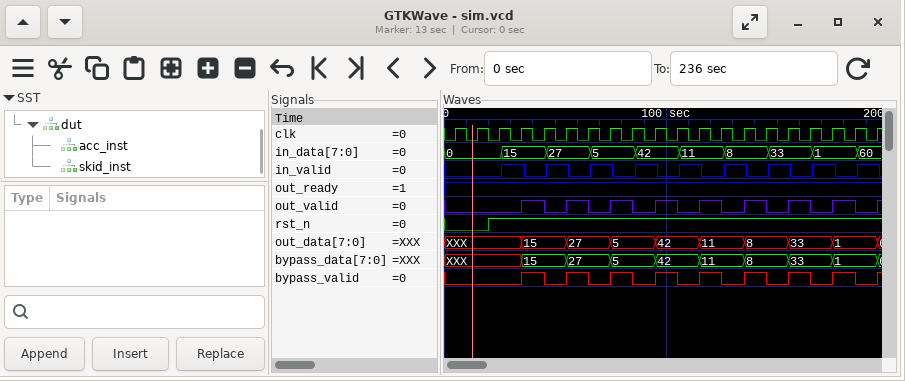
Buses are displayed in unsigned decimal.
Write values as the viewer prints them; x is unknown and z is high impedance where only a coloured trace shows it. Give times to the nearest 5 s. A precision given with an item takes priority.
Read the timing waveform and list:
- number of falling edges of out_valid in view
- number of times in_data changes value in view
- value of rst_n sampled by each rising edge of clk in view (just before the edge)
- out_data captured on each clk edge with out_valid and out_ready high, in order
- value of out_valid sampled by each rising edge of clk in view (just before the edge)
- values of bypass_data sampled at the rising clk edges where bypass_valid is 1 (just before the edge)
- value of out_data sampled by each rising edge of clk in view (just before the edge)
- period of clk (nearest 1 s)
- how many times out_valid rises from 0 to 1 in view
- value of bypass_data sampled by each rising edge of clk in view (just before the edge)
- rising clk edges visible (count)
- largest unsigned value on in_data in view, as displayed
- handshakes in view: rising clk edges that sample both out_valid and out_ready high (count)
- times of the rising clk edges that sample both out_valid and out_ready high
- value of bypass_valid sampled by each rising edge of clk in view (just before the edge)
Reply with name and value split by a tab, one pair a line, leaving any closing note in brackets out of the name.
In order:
number of falling edges of out_valid in view	8
number of times in_data changes value in view	9
value of rst_n sampled by each rising edge of clk in view	0 0 1 1 1 1 1 1 1 1 1 1 1 1 1 1 1 1 1 1
out_data captured on each clk edge with out_valid and out_ready high, in order	15, 27, 5, 42, 11, 8, 33, 1
value of out_valid sampled by each rising edge of clk in view	0 0 0 0 1 0 1 0 1 0 1 0 1 0 1 0 1 0 1 0
values of bypass_data sampled at the rising clk edges where bypass_valid is 1	15, 27, 5, 42, 11, 8, 33, 1
value of out_data sampled by each rising edge of clk in view	XXX, XXX, XXX, XXX, 15, 15, 27, 27, 5, 5, 42, 42, 11, 11, 8, 8, 33, 33, 1, 1
period of clk	10 s
how many times out_valid rises from 0 to 1 in view	9
value of bypass_data sampled by each rising edge of clk in view	XXX, XXX, XXX, XXX, 15, 15, 27, 27, 5, 5, 42, 42, 11, 11, 8, 8, 33, 33, 1, 1
rising clk edges visible	20
largest unsigned value on in_data in view, as displayed	60
handshakes in view: rising clk edges that sample both out_valid and out_ready high	8
times of the rising clk edges that sample both out_valid and out_ready high	45 s, 65 s, 85 s, 105 s, 125 s, 145 s, 165 s, 185 s
value of bypass_valid sampled by each rising edge of clk in view	0 0 0 0 1 0 1 0 1 0 1 0 1 0 1 0 1 0 1 0
